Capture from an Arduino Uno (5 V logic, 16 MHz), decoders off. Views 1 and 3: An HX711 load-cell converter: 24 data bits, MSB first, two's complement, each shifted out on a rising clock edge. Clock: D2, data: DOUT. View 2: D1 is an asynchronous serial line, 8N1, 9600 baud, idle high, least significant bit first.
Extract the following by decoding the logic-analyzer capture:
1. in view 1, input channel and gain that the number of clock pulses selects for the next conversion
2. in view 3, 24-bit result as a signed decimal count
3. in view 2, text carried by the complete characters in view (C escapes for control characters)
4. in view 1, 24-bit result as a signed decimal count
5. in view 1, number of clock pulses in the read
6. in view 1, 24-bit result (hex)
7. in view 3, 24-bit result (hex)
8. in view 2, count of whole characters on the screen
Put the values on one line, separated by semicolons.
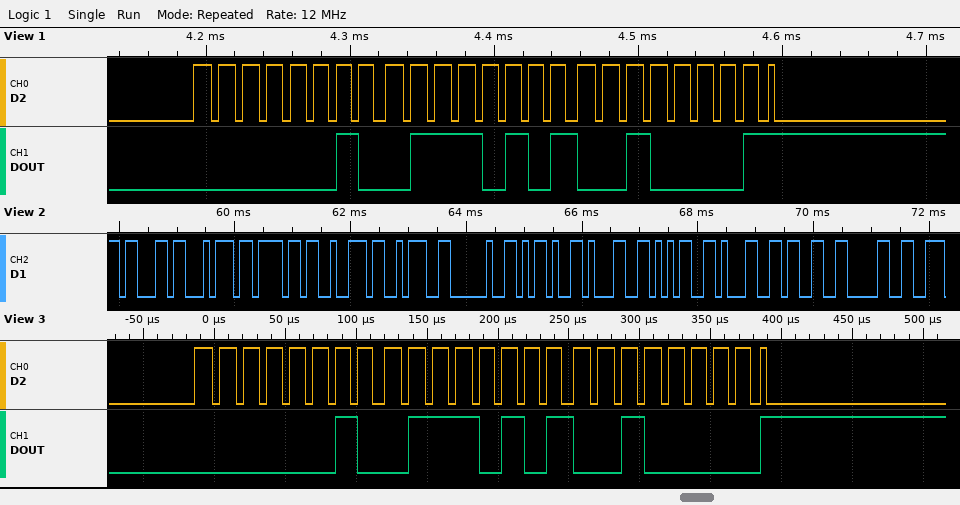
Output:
channel A, gain 128; 161056; "ctor: -15130"; 161057; 25; 0x027521; 0x027520; 12
